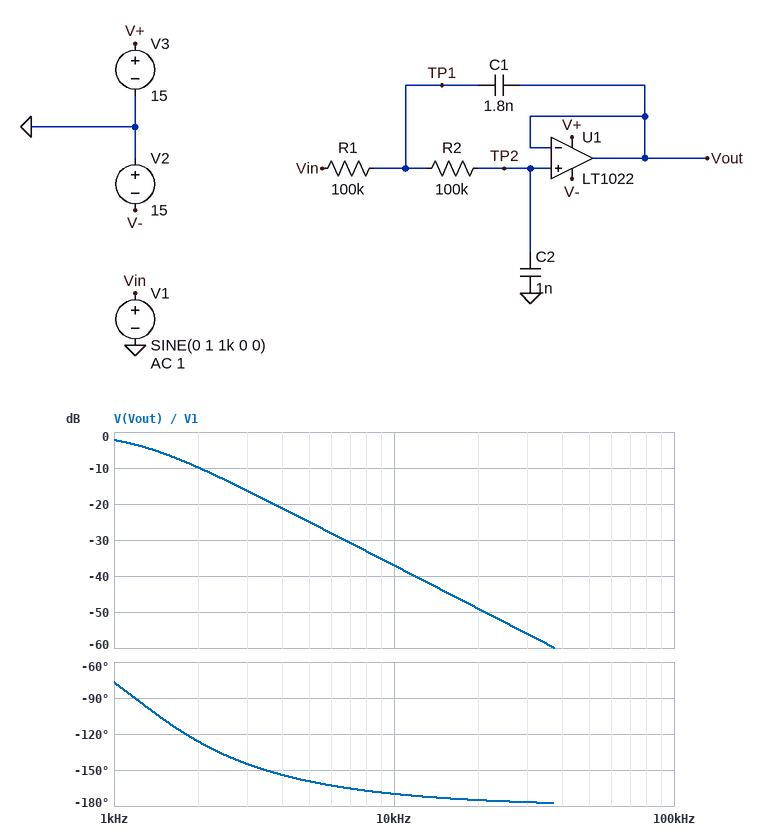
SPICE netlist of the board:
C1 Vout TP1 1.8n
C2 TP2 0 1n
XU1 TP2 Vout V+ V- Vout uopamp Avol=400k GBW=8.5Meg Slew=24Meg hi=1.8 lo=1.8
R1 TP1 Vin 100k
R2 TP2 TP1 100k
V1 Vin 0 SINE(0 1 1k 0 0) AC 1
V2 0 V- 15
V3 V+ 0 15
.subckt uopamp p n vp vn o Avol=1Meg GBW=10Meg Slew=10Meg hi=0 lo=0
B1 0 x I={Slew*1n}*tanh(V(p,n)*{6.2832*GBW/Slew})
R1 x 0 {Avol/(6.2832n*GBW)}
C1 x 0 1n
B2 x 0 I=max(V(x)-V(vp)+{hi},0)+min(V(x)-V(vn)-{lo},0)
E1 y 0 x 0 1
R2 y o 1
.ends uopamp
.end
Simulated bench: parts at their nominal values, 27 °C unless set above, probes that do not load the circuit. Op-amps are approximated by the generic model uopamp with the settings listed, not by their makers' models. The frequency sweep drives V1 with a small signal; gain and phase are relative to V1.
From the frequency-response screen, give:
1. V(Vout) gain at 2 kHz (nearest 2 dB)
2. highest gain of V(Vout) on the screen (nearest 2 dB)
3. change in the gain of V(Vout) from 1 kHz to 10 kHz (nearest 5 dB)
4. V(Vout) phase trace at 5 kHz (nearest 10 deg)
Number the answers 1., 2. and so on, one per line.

1. -10 dB
2. -2 dB
3. -35 dB
4. -160 deg
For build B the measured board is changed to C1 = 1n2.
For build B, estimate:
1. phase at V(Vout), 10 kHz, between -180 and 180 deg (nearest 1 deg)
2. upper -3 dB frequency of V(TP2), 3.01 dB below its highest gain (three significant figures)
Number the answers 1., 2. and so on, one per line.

1. -165 deg
2. 1.06 kHz
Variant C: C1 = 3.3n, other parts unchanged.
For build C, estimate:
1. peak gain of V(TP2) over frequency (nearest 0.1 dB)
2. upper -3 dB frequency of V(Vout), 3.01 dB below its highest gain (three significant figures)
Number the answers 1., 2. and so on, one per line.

1. 0.7 dB
2. 1.00 kHz
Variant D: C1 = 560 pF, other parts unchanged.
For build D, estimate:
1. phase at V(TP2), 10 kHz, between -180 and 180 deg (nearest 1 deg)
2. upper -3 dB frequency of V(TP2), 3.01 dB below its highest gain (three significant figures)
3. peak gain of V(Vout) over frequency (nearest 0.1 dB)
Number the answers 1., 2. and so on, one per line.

1. -149 deg
2. 921 Hz
3. 0 dB
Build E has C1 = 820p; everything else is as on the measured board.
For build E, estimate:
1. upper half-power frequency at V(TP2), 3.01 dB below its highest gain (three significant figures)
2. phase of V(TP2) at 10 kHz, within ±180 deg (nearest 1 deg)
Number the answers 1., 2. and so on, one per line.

1. 984 Hz
2. -158 deg
